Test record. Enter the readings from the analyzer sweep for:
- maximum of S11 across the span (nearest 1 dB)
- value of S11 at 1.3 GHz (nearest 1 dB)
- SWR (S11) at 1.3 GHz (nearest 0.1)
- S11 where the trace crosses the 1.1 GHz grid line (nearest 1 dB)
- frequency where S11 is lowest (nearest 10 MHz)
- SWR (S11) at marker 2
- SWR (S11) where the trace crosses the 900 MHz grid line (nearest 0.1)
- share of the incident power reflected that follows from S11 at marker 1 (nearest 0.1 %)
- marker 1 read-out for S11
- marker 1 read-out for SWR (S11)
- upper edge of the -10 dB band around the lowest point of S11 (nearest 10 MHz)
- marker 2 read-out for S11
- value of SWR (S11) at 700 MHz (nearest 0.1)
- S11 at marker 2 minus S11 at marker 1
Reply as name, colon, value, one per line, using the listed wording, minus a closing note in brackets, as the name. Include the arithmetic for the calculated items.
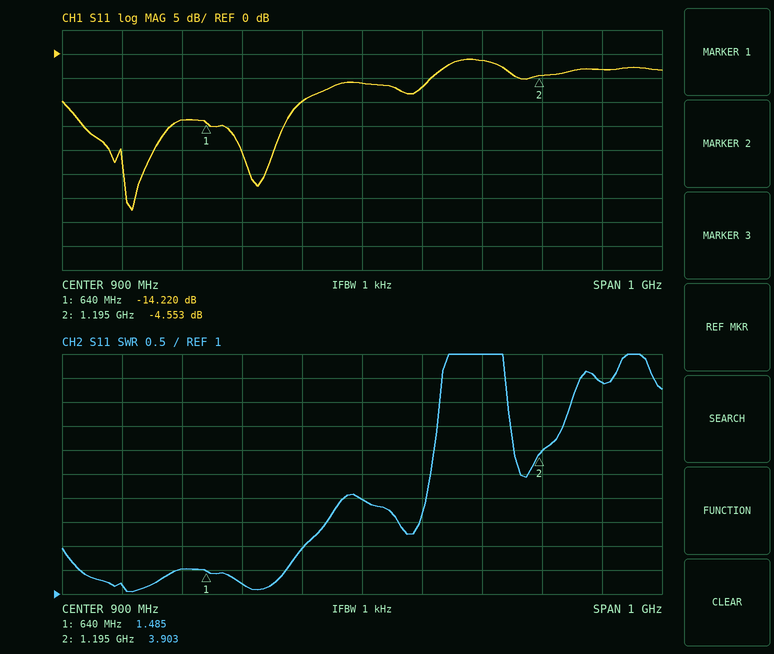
maximum of S11 across the span: -1 dB
value of S11 at 1.3 GHz: -3 dB
SWR (S11) at 1.3 GHz: 5.4
S11 where the trace crosses the 1.1 GHz grid line: -1 dB
frequency where S11 is lowest: 520 MHz
SWR (S11) at marker 2: 3.903
SWR (S11) where the trace crosses the 900 MHz grid line: 3.0
share of the incident power reflected that follows from S11 at marker 1: 10^(-14.22/10) ≈ 3.8 %
marker 1 read-out for S11: -14.220 dB
marker 1 read-out for SWR: 1.485
upper edge of the -10 dB band around the lowest point of S11: 800 MHz
marker 2 read-out for S11: -4.553 dB
value of SWR (S11) at 700 MHz: 1.2
S11 at marker 2 minus S11 at marker 1: -4.553 − (-14.22) = 9.667 dB
